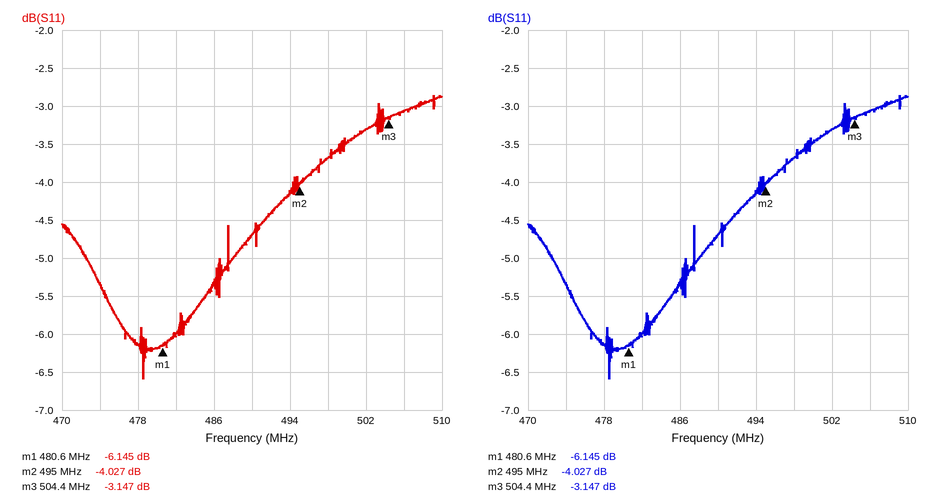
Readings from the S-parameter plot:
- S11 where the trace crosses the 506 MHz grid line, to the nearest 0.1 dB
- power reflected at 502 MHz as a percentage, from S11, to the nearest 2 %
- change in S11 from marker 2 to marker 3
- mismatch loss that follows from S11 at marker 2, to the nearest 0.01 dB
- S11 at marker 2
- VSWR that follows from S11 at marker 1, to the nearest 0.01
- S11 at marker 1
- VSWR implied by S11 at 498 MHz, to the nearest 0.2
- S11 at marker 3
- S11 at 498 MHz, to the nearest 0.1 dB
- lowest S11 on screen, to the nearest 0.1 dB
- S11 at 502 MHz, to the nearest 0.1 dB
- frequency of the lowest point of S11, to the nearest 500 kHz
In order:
-3.1 dB
46 %
0.880 dB
2.19 dB
-4.027 dB
2.94
-6.145 dB
4.8
-3.147 dB
-3.7 dB
-6.6 dB
-3.3 dB
478.5 MHz
